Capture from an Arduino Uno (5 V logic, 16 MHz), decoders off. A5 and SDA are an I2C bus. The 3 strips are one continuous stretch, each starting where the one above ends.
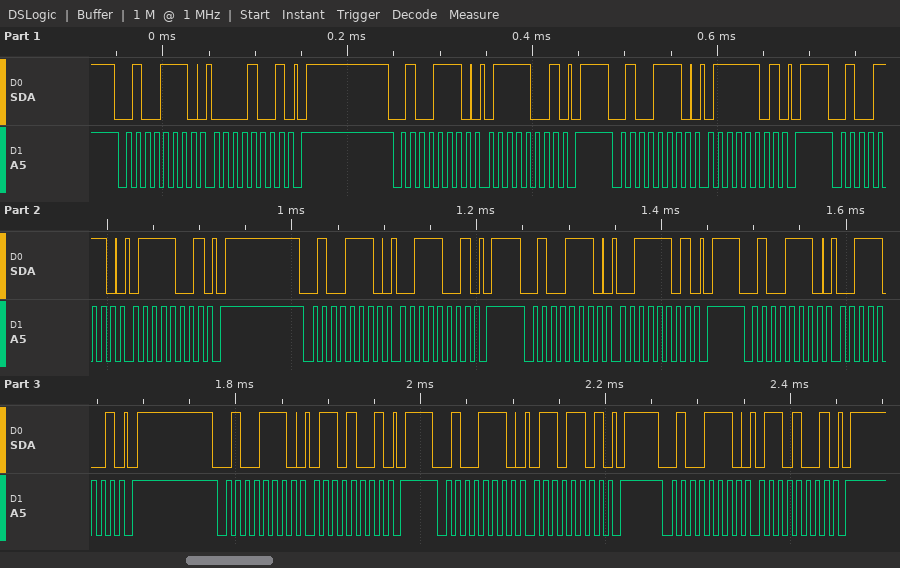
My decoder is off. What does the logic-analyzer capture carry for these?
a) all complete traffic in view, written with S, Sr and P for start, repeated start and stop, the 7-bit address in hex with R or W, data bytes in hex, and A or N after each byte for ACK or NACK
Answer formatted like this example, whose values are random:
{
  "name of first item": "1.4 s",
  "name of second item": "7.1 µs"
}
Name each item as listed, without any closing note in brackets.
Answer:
{
  "all complete traffic in view, written with S, Sr and P for start, repeated start and stop, the 7-bit address in hex with R or W, data bytes in hex, and A or N after each byte for ACK or NACK": "S 27W A 09 A P S 27W A 79 A P S 27W A 7D A P S 27W A 79 A P S 27W A 39 A P S 27W A 3D A P S 27W A 39 A P S 27W A 69 A P S 27W A 6D A P S 27W A 69 A P"
}
